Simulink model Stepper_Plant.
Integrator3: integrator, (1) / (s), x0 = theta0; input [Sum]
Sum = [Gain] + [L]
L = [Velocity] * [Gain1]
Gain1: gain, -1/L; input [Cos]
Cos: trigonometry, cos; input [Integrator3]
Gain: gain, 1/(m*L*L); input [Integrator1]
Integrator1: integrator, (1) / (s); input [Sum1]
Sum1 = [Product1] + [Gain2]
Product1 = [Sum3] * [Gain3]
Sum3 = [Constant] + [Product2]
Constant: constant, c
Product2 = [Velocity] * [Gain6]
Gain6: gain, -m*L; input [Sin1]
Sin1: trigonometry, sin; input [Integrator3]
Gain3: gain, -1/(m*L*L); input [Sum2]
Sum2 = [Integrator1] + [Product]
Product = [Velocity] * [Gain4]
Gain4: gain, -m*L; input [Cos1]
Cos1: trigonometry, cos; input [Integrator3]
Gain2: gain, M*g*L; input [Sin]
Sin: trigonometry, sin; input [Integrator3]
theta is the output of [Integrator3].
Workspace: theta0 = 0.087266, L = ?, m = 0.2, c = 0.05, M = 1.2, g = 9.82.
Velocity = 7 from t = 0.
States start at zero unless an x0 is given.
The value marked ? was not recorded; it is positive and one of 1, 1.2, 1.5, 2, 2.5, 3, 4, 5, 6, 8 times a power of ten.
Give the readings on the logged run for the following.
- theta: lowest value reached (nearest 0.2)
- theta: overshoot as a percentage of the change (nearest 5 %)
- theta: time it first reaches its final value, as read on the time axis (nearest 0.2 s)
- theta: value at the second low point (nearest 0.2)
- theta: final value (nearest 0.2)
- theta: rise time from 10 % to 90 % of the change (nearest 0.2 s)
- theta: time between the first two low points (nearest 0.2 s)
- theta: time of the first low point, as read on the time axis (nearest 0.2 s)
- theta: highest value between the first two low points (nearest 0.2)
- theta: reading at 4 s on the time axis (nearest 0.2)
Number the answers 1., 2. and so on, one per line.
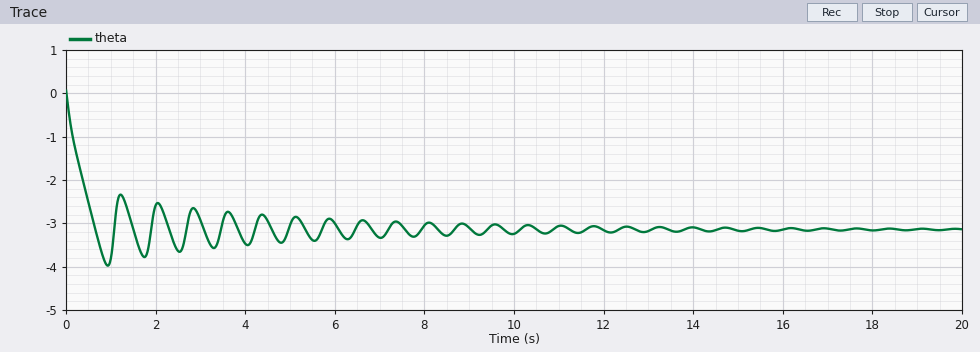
1. -4.0
2. 25 %
3. 0.6 s
4. -3.8
5. -3.2
6. 0.6 s
7. 0.8 s
8. 1.0 s
9. -2.4
10. -3.4
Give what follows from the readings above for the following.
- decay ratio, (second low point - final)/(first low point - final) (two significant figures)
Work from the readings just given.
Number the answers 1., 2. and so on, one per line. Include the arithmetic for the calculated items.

1. (-3.8 - (-3.2)) / (-4 - (-3.2)) = 0.75
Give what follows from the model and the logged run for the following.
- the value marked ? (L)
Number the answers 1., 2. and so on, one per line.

1. 0.8
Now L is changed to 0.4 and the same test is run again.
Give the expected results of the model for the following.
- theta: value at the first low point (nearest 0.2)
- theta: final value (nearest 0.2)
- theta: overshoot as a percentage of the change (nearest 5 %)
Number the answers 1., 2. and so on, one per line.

1. -3.6
2. -3.2
3. 10 %
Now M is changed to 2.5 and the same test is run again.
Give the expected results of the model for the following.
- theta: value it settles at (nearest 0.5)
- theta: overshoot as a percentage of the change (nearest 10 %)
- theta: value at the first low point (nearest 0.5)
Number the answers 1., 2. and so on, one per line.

1. -3.0
2. 40 %
3. -4.5
